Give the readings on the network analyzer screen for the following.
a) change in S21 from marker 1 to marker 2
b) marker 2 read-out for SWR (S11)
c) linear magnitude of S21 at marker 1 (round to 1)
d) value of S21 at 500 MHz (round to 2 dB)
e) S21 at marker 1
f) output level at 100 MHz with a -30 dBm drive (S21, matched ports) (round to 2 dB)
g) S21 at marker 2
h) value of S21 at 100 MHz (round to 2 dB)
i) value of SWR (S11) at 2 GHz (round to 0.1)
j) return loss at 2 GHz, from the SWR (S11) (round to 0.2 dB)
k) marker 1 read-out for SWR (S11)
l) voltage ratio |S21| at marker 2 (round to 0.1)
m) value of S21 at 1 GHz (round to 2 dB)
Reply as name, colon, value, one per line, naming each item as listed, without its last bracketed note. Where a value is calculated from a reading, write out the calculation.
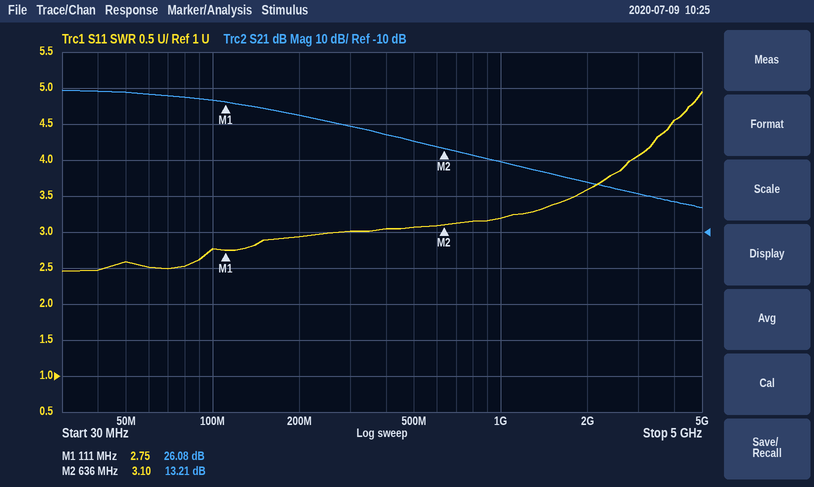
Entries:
change in S21 from marker 1 to marker 2: 13.21 − (26.08) = -12.87 dB
marker 2 read-out for SWR: 3.10
linear magnitude of S21 at marker 1: 10^(26.08/20) ≈ 20
value of S21 at 500 MHz: 16 dB
S21 at marker 1: 26.08 dB
output level at 100 MHz with a -30 dBm drive (S21, matched ports): -30 dBm + (26 dB) = -4 dBm
S21 at marker 2: 13.21 dB
value of S21 at 100 MHz: 26 dB
value of SWR (S11) at 2 GHz: 3.6
return loss at 2 GHz, from the SWR (S11): −20 log10((3.6 − 1)/(3.6 + 1)) ≈ 5.0 dB
marker 1 read-out for SWR: 2.75
voltage ratio |S21| at marker 2: 10^(13.21/20) ≈ 4.6
value of S21 at 1 GHz: 10 dB
